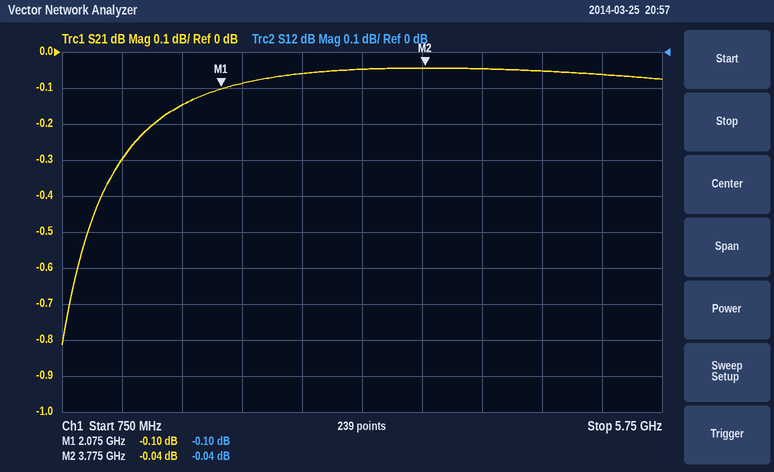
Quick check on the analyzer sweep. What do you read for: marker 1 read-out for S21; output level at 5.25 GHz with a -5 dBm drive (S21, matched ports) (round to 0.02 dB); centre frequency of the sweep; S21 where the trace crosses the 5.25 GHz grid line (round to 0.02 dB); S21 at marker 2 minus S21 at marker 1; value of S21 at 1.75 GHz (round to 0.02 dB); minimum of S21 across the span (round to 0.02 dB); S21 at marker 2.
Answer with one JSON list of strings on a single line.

["-0.10 dB", "-5.06 dBm", "3.25 GHz", "-0.06 dB", "0.06 dB", "-0.14 dB", "-0.82 dB", "-0.04 dB"]
